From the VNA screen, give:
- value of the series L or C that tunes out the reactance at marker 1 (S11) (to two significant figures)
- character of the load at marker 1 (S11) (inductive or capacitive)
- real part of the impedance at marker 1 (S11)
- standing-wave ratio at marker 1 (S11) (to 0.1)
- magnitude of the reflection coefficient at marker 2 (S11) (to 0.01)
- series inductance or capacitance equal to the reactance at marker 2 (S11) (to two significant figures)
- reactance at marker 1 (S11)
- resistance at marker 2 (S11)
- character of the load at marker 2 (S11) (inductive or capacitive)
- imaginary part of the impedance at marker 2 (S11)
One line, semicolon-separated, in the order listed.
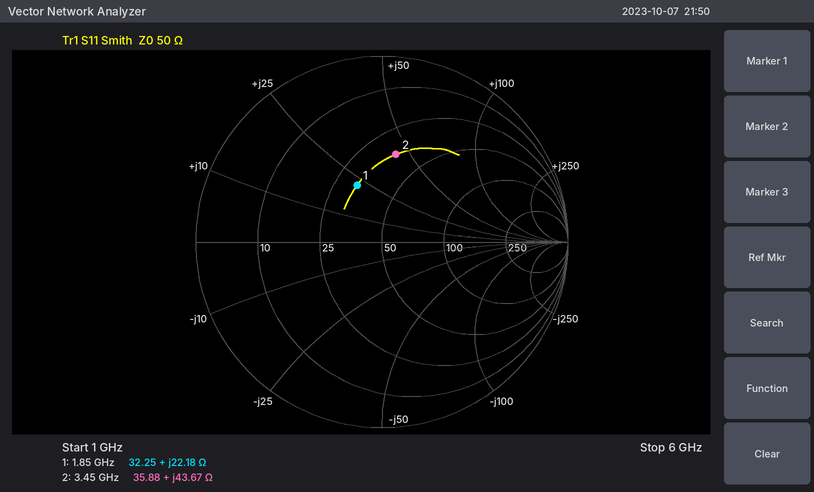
3.9 pF; inductive; 32.25 Ω; 2.0; 0.48; 2.0 nH; +22.18 Ω; 35.88 Ω; inductive; +43.67 Ω
